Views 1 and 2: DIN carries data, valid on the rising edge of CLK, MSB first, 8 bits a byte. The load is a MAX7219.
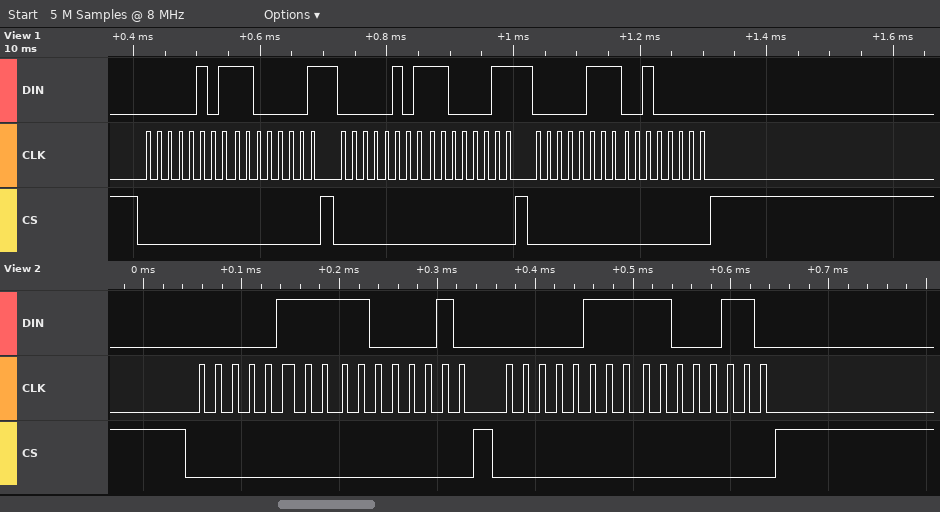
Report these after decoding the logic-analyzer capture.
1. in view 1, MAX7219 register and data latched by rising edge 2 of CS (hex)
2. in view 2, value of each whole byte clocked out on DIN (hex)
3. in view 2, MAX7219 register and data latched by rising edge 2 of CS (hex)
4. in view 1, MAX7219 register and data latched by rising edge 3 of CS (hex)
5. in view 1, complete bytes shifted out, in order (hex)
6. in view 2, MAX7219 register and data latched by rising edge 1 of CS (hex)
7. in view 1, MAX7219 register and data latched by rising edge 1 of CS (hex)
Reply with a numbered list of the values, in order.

1. register 0x5, data 0xC3
2. 07 C2 07 C6
3. register 0x7, data 0xC6
4. register 0x7, data 0x20
5. 0x05 0xC1 0x05 0xC3 0x07 0x20
6. register 0x7, data 0xC2
7. register 0x5, data 0xC1
